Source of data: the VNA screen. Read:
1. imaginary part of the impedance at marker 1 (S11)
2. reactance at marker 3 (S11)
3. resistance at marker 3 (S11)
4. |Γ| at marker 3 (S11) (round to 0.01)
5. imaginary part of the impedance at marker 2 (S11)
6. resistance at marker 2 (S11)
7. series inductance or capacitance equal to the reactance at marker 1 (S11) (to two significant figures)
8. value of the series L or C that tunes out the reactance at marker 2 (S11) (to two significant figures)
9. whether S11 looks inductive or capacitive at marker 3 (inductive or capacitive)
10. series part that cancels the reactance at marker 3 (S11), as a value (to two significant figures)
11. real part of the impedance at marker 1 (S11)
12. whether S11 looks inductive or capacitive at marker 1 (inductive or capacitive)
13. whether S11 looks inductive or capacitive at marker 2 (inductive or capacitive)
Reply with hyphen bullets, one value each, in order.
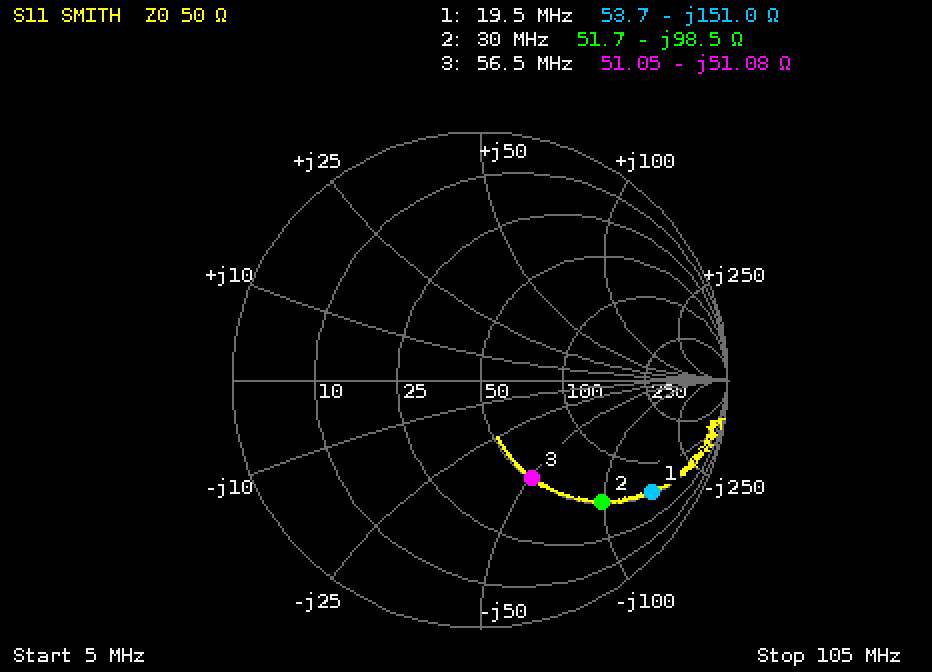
- -151.0 Ω
- -51.08 Ω
- 51.05 Ω
- 0.45
- -98.5 Ω
- 51.7 Ω
- 54 pF
- 520 nH
- capacitive
- 140 nH
- 53.7 Ω
- capacitive
- capacitive
